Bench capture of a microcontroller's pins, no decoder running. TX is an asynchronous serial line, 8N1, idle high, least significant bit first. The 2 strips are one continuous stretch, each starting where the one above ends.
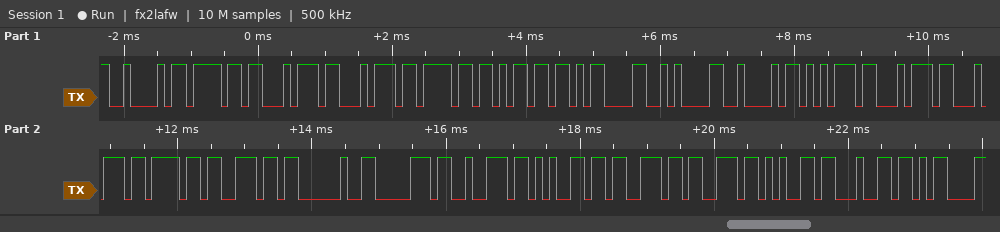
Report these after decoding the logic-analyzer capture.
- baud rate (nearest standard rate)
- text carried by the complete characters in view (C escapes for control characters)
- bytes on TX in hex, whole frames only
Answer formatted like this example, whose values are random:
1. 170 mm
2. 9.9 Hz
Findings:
1. 9600 baud
2. "Bottom\r\nButton pressed\r"
3. 42 6F 74 74 6F 6D 0D 0A 42 75 74 74 6F 6E 20 70 72 65 73 73 65 64 0D
